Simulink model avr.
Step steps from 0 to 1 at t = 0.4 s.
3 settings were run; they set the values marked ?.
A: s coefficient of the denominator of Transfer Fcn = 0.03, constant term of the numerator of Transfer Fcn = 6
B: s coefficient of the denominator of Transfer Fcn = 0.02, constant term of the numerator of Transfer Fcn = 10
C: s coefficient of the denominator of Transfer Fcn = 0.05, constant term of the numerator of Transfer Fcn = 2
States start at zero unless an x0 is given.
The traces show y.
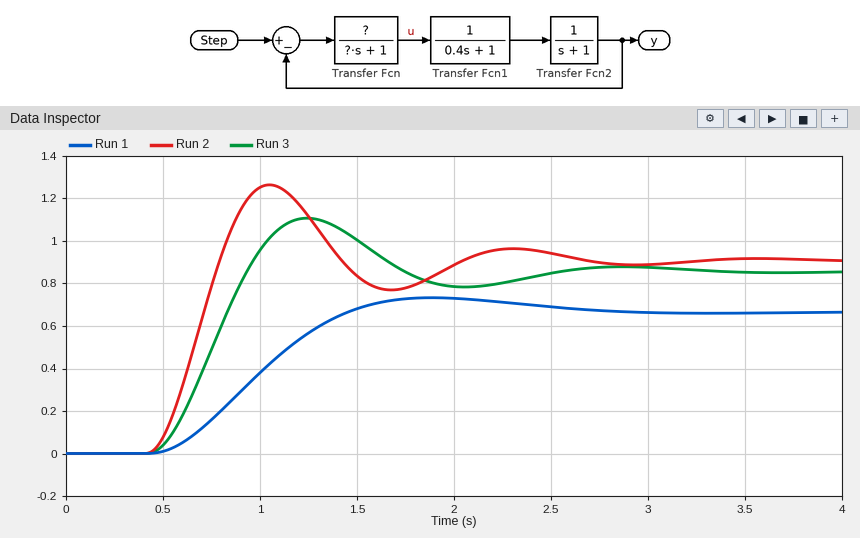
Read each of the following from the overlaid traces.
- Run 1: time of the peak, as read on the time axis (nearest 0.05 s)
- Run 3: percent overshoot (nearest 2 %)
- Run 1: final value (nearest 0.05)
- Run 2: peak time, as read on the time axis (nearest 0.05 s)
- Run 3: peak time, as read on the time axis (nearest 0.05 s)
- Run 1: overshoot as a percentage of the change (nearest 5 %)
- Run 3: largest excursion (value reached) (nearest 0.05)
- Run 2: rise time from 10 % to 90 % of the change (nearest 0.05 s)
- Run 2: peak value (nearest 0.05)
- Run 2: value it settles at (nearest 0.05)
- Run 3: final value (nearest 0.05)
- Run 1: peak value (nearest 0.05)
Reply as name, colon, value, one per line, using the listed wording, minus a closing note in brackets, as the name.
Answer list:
Run 1: time of the peak, as read on the time axis: 1.90 s
Run 3: percent overshoot: 30 %
Run 1: final value: 0.65
Run 2: peak time, as read on the time axis: 1.05 s
Run 3: peak time, as read on the time axis: 1.25 s
Run 1: overshoot as a percentage of the change: 10 %
Run 3: largest excursion (value reached): 1.10
Run 2: rise time from 10 % to 90 % of the change: 0.25 s
Run 2: peak value: 1.25
Run 2: value it settles at: 0.90
Run 3: final value: 0.85
Run 1: peak value: 0.75
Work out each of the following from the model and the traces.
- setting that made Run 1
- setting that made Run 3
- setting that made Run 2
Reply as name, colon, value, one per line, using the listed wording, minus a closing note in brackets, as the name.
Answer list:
setting that made Run 1: C
setting that made Run 3: A
setting that made Run 2: B
